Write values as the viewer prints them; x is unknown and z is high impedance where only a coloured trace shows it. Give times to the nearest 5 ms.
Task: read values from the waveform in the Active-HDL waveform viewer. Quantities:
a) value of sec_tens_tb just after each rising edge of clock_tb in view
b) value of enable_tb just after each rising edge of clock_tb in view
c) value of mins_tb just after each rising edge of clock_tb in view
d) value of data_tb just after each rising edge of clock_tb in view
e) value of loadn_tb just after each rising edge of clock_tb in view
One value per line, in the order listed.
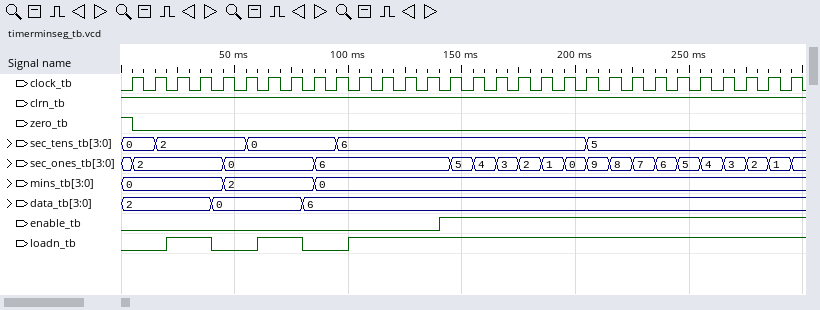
0, 2, 2, 2, 2, 0, 0, 0, 0, 6, 6, 6, 6, 6, 6, 6, 6, 6, 6, 6, 5, 5, 5, 5, 5, 5, 5, 5, 5, 5
0 0 0 0 0 0 0 0 0 0 0 0 0 0 1 1 1 1 1 1 1 1 1 1 1 1 1 1 1 1
0, 0, 0, 0, 2, 2, 2, 2, 0, 0, 0, 0, 0, 0, 0, 0, 0, 0, 0, 0, 0, 0, 0, 0, 0, 0, 0, 0, 0, 0
2, 2, 2, 2, 0, 0, 0, 0, 6, 6, 6, 6, 6, 6, 6, 6, 6, 6, 6, 6, 6, 6, 6, 6, 6, 6, 6, 6, 6, 6
0 0 1 1 0 0 1 1 0 0 1 1 1 1 1 1 1 1 1 1 1 1 1 1 1 1 1 1 1 1
